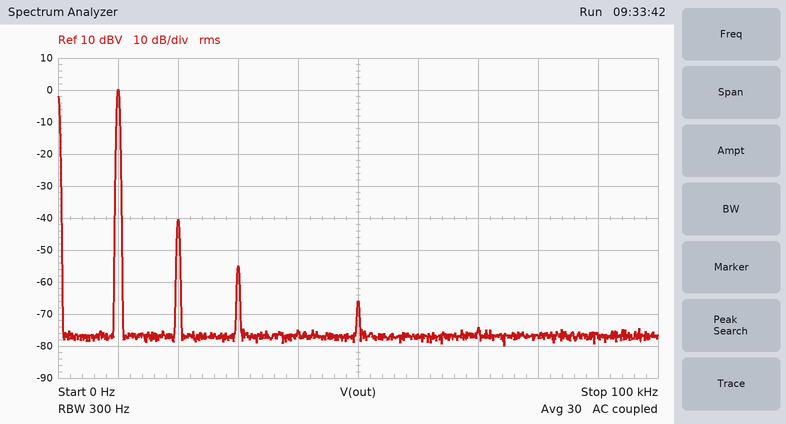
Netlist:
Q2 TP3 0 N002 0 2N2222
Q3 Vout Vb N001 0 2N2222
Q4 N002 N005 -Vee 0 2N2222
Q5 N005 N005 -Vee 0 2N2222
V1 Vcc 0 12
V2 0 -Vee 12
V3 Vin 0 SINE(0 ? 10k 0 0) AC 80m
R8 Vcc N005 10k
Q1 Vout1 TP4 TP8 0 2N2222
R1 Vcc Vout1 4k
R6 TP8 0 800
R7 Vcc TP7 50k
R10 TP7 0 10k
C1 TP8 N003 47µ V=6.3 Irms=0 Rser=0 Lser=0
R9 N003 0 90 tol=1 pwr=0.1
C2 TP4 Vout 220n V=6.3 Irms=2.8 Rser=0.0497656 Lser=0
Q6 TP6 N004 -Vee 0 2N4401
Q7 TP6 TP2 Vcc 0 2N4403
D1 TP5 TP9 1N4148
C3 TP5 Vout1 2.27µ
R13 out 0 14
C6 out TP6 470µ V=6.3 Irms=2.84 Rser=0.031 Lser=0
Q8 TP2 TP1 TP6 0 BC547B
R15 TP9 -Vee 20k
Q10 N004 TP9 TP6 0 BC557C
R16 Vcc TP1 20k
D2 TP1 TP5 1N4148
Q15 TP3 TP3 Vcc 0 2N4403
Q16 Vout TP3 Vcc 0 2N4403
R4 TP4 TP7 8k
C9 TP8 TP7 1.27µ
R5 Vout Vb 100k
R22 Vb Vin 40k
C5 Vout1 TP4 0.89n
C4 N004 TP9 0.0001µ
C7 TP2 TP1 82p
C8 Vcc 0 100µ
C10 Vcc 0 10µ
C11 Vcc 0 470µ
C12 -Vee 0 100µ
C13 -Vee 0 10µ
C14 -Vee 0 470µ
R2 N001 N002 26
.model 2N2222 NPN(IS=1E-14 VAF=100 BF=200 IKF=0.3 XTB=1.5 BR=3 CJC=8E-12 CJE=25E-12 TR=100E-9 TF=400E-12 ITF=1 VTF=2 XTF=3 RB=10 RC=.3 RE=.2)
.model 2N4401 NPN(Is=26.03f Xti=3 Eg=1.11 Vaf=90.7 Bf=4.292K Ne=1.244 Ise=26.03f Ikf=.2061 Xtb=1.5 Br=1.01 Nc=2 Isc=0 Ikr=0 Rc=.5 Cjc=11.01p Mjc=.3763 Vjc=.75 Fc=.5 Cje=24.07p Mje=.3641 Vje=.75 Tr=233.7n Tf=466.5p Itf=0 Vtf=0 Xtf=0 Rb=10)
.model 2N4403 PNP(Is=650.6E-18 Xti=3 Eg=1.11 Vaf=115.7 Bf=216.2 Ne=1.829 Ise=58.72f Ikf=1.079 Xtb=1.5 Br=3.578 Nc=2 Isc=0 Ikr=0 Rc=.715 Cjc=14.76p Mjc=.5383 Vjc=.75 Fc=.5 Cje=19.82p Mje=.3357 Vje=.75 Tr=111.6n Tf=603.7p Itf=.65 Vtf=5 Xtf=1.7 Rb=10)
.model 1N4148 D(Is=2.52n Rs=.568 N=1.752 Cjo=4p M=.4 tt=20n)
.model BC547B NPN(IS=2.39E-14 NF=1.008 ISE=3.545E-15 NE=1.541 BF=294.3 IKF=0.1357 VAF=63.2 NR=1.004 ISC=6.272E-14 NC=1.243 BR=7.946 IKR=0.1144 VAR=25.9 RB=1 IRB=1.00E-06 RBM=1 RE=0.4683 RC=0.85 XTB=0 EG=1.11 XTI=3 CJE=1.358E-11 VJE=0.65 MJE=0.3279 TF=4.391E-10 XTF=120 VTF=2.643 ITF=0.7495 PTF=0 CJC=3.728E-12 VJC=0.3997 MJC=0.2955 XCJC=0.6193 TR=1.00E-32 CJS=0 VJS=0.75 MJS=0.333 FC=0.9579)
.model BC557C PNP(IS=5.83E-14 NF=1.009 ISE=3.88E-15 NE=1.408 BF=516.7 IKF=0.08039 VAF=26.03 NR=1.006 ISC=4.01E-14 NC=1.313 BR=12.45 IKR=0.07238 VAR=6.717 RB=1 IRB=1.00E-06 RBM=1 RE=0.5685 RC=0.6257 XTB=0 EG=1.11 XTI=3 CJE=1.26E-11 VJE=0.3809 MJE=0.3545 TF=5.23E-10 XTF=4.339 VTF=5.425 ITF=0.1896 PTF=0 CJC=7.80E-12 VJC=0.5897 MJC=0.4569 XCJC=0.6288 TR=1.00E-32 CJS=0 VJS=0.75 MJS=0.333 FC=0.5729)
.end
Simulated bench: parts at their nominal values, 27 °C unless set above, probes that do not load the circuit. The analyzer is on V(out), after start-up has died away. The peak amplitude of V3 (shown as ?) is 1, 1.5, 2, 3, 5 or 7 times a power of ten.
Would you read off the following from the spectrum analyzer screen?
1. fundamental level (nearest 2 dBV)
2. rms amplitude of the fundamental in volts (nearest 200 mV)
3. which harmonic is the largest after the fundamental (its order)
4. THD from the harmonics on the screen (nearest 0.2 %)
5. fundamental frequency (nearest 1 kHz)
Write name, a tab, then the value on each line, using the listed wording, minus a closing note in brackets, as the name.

fundamental level	0 dBV
rms amplitude of the fundamental in volts	1.0 V
which harmonic is the largest after the fundamental	2
THD from the harmonics on the screen	1.0 %
fundamental frequency	10 kHz
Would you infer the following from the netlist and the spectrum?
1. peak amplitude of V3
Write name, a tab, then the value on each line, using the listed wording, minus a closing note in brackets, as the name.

peak amplitude of V3	30 mV
